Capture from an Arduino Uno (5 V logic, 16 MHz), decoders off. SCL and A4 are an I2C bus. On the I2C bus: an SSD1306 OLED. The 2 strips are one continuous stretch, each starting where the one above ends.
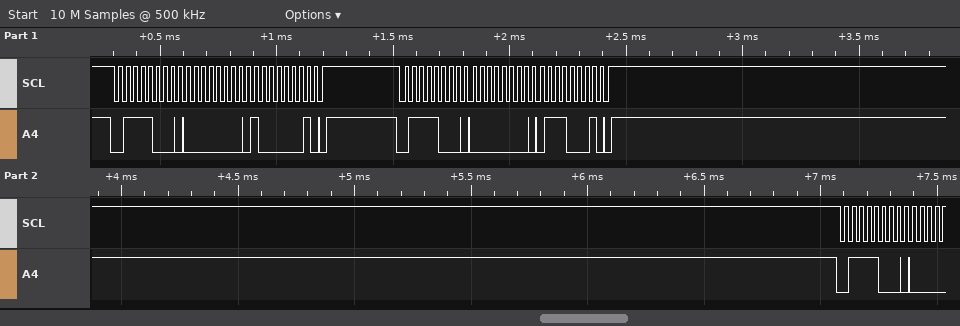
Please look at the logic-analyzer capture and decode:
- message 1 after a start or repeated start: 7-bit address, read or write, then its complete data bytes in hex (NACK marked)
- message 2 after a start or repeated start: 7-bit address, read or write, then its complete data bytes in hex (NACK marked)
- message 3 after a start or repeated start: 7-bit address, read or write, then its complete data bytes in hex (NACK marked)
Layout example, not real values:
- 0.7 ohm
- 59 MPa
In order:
- 0x3C write: 00 81
- 0x3C write: 00 71
- 0x3C write
